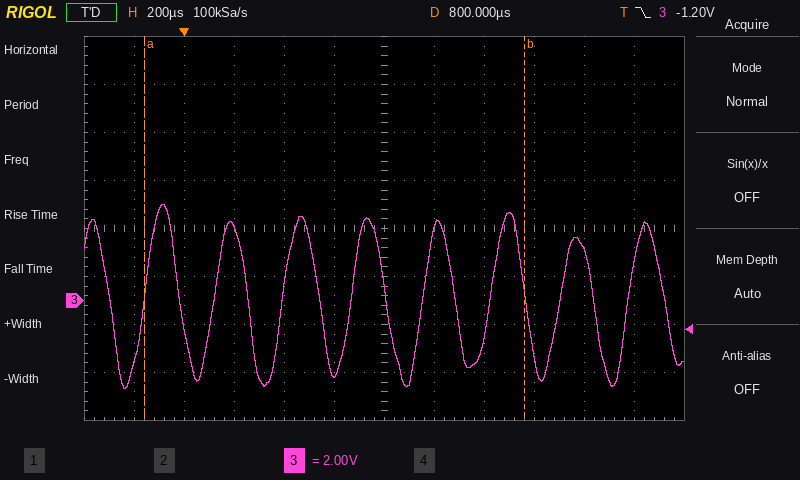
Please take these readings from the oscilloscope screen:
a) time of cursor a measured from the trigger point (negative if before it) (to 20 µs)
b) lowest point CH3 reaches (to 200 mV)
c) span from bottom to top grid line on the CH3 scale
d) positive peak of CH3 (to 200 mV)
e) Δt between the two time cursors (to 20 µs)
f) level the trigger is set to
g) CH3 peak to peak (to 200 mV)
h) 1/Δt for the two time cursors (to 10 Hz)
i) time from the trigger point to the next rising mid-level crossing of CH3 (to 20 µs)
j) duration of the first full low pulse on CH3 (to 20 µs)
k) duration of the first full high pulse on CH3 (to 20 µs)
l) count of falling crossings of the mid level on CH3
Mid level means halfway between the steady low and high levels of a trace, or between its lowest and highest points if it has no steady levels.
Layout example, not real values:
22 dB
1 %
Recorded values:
-160 µs
-3.6 V
16 V
4.0 V
1.52 ms
-1.20 V
7.6 V
660 Hz
120 µs
140 µs
140 µs
9
